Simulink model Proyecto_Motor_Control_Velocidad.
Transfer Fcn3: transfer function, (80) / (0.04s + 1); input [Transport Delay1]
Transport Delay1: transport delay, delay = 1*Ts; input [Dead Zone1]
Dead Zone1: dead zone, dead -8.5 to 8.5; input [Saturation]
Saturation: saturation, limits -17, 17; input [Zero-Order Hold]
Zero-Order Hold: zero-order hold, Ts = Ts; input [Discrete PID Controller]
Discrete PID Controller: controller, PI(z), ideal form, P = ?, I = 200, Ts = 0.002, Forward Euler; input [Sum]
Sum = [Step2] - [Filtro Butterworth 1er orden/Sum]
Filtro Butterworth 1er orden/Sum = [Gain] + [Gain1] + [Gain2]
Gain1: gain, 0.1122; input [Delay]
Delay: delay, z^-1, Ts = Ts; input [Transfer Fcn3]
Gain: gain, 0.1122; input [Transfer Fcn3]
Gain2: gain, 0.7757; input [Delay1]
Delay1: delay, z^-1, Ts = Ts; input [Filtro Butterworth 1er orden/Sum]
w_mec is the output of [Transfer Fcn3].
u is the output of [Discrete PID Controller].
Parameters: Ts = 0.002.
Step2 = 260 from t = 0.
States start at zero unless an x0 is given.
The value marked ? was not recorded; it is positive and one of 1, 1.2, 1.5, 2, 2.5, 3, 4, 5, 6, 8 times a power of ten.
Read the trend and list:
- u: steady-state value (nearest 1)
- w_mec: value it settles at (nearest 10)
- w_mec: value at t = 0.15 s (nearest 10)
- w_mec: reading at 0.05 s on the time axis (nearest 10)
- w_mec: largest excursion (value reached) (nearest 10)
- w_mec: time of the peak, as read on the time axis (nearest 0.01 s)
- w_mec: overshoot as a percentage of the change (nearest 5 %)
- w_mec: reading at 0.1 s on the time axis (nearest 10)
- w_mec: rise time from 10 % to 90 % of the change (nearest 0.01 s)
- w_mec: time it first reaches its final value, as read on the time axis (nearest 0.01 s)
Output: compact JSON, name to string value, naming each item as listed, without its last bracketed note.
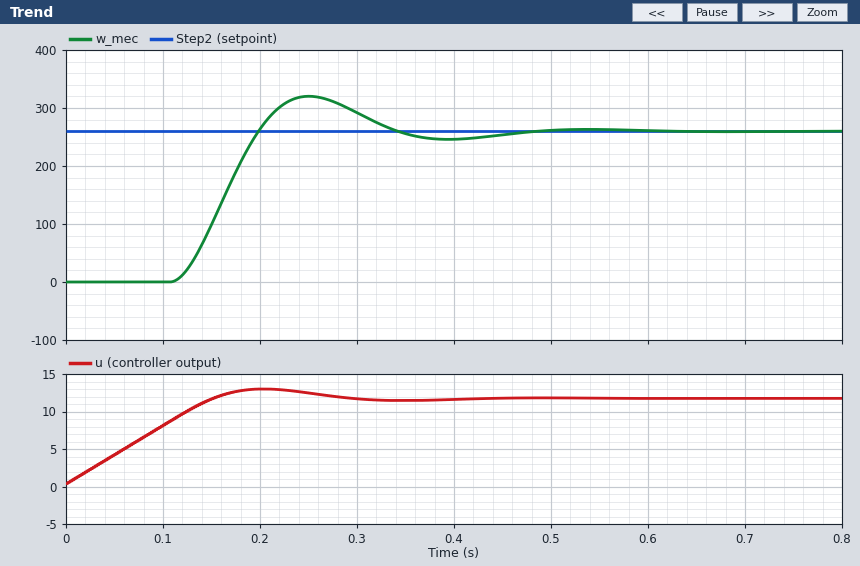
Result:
{"u: steady-state value": "12", "w_mec: value it settles at": "260", "w_mec: value at t = 0.15 s": "100", "w_mec: reading at 0.05 s on the time axis": "0", "w_mec: largest excursion (value reached)": "320", "w_mec: time of the peak, as read on the time axis": "0.25 s", "w_mec: overshoot as a percentage of the change": "25 %", "w_mec: reading at 0.1 s on the time axis": "0", "w_mec: rise time from 10 % to 90 % of the change": "0.06 s", "w_mec: time it first reaches its final value, as read on the time axis": "0.20 s"}
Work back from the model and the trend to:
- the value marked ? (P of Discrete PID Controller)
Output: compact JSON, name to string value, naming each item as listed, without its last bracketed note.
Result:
{"the value marked ?": "0.0015"}
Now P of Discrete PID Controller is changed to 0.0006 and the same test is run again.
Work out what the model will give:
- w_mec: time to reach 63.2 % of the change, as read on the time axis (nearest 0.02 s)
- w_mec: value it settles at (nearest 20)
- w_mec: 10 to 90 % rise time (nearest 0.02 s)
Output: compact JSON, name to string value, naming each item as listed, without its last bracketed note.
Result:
{"w_mec: time to reach 63.2 % of the change, as read on the time axis": "0.38 s", "w_mec: value it settles at": "260", "w_mec: 10 to 90 % rise time": "0.14 s"}
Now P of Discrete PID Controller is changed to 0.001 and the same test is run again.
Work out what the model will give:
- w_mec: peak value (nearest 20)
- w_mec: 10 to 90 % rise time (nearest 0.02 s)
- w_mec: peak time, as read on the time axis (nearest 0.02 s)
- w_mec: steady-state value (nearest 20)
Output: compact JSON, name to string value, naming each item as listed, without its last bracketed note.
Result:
{"w_mec: peak value": "300", "w_mec: 10 to 90 % rise time": "0.08 s", "w_mec: peak time, as read on the time axis": "0.36 s", "w_mec: steady-state value": "260"}
